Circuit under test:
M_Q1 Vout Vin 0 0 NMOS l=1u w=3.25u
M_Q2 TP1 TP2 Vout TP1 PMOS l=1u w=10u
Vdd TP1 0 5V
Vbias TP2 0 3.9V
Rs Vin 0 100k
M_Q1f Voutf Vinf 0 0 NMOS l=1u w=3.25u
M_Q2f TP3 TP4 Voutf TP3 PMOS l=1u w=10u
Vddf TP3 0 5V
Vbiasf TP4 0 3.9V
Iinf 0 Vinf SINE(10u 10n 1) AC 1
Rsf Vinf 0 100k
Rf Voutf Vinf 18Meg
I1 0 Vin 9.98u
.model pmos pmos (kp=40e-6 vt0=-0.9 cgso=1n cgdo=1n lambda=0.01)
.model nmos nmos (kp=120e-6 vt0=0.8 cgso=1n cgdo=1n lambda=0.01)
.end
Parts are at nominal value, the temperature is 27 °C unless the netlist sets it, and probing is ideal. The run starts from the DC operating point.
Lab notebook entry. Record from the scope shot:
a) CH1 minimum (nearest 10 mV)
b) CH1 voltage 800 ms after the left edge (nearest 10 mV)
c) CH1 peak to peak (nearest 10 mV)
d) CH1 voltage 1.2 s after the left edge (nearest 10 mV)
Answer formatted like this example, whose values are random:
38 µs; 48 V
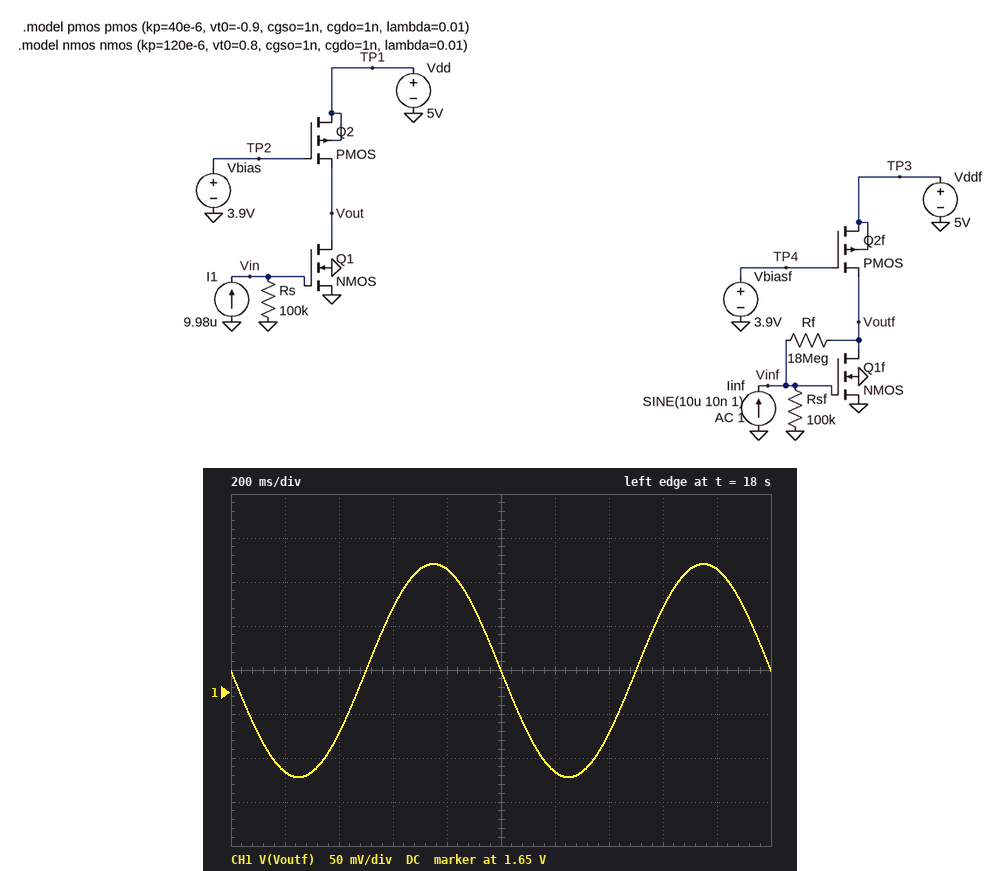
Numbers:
1.55 V; 1.79 V; 240 mV; 1.56 V
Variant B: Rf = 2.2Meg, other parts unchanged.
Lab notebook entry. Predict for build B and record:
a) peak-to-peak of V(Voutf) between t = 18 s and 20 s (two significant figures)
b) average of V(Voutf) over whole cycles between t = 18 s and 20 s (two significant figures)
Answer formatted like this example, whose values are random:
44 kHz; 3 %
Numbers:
37 mV; 1.1 V
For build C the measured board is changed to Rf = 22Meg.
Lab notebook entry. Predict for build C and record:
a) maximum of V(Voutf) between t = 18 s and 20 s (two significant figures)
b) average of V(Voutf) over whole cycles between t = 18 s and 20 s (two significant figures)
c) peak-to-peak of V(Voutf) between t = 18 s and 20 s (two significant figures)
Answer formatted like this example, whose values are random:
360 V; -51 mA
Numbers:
1.9 V; 1.8 V; 280 mV
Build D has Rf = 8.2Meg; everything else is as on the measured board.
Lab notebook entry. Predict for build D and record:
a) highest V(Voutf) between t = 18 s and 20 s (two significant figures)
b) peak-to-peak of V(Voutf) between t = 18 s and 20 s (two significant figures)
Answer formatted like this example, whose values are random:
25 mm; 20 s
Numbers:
1.4 V; 130 mV
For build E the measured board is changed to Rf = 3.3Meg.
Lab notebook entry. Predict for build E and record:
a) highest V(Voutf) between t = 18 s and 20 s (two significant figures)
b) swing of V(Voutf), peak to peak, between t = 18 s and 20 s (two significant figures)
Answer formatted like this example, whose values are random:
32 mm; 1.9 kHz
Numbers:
1.2 V; 55 mV
